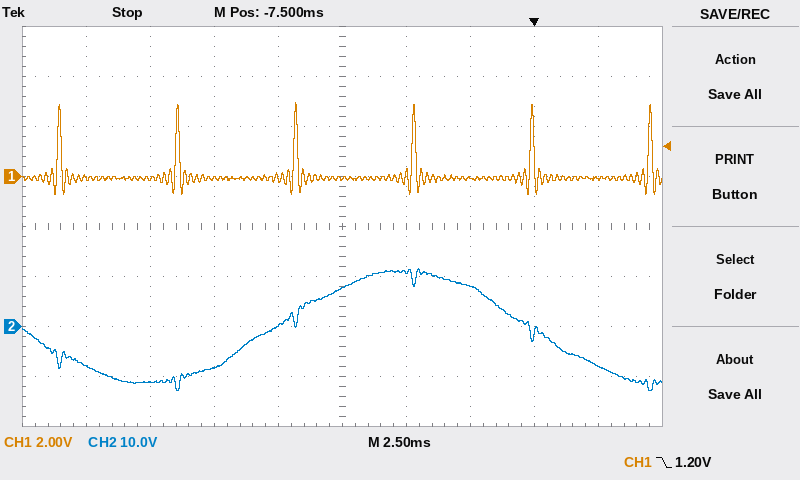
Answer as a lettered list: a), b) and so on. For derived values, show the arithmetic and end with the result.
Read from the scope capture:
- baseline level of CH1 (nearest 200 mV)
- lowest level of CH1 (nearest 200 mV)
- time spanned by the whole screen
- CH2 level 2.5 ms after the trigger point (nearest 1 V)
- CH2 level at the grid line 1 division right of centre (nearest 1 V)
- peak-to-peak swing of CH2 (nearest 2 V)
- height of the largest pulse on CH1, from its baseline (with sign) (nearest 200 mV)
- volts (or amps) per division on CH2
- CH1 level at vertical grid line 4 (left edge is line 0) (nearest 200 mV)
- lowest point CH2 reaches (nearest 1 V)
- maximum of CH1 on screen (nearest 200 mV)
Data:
a) 0.0 V
b) -800 mV
c) 25 ms
d) -8 V
e) 11 V
f) 24 V
g) 3.0 V − (0.0 V) = +3.0 V
h) 10 V
i) 0.0 V
j) -13 V
k) 3.0 V
